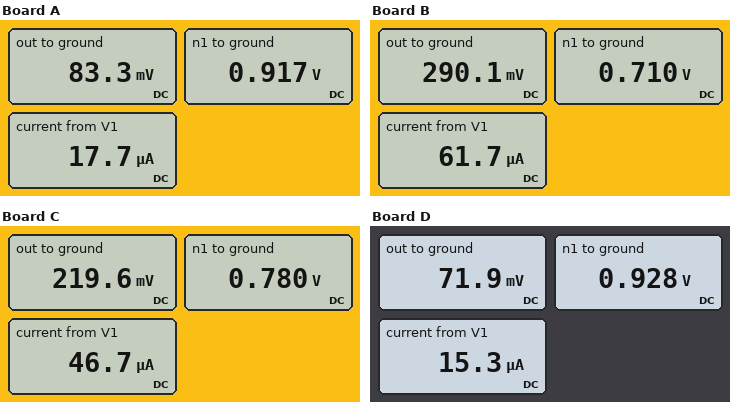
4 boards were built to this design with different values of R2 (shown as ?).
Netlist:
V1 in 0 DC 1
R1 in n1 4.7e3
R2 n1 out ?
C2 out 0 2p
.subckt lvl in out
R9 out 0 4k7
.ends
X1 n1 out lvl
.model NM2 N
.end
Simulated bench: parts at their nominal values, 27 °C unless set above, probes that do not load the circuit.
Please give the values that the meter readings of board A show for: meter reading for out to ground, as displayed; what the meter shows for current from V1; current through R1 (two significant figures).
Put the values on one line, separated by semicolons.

83.3 mV; 17.7 µA; 18 µA
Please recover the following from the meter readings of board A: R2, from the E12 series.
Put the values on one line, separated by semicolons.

47 kΩ
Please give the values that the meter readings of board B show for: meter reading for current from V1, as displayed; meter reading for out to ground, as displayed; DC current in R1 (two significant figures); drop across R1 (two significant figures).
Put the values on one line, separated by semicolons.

61.7 µA; 290.1 mV; 62 µA; 290 mV
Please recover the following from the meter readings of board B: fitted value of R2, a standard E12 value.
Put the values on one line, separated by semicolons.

6.8 kΩ
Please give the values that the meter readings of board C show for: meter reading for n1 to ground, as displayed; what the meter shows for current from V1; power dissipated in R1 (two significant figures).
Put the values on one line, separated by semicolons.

0.780 V; 46.7 µA; 10 µW
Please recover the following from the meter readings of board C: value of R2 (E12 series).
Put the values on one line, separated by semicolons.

12 kΩ
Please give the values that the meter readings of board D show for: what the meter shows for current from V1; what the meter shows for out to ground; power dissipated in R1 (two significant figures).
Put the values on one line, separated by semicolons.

15.3 µA; 71.9 mV; 1.1 µW
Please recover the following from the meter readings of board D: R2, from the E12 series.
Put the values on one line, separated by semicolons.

56 kΩ
